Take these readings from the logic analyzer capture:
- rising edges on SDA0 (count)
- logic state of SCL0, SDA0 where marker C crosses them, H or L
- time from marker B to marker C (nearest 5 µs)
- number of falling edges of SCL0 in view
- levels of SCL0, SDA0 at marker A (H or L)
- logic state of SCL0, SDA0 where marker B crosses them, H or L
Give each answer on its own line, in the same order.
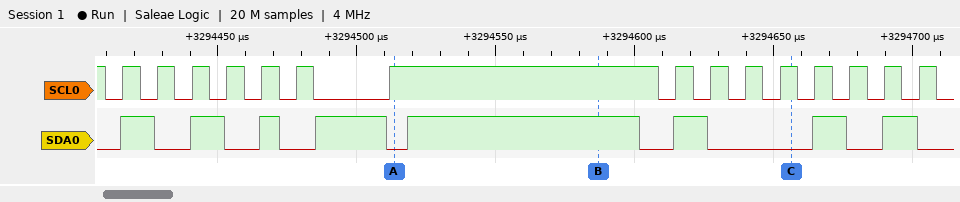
8
SCL0=H, SDA0=L
70 µs
16
SCL0=H, SDA0=L
SCL0=H, SDA0=H
